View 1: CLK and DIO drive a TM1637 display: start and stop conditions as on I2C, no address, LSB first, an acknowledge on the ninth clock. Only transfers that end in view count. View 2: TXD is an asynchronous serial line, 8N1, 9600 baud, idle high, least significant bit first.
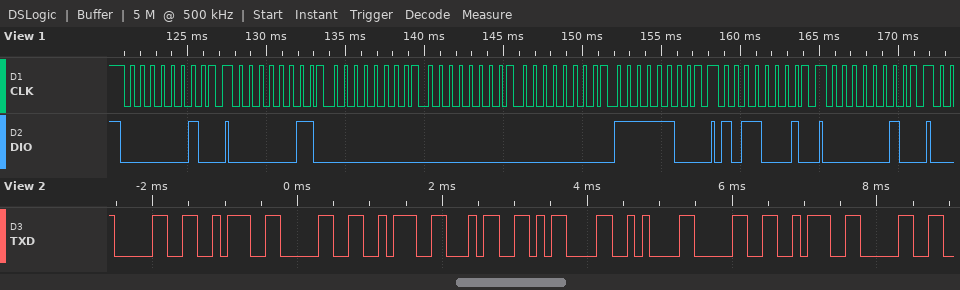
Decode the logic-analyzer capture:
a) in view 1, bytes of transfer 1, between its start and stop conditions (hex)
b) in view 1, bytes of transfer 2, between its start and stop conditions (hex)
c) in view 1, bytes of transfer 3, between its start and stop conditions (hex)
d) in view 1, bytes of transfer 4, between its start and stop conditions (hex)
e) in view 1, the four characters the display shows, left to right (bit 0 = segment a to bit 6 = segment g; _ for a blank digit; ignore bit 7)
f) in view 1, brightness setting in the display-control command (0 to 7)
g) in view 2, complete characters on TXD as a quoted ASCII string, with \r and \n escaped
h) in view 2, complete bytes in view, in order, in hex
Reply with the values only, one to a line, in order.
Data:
40
C0 00 00 00 3F
8D
40
___0
5
"0:0:4\r\n0:0"
30 3A 30 3A 34 0D 0A 30 3A 30
